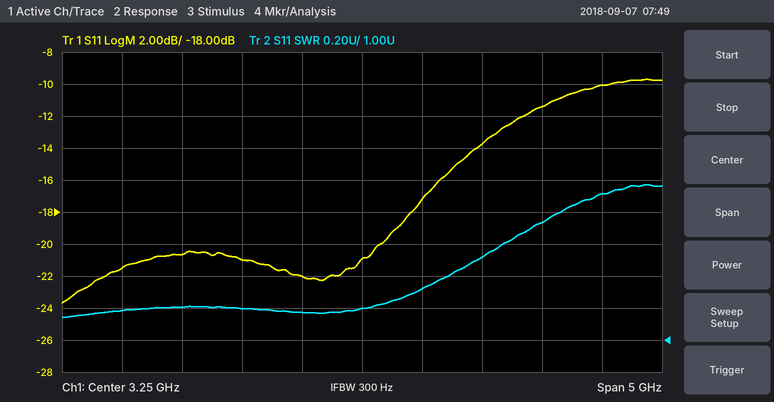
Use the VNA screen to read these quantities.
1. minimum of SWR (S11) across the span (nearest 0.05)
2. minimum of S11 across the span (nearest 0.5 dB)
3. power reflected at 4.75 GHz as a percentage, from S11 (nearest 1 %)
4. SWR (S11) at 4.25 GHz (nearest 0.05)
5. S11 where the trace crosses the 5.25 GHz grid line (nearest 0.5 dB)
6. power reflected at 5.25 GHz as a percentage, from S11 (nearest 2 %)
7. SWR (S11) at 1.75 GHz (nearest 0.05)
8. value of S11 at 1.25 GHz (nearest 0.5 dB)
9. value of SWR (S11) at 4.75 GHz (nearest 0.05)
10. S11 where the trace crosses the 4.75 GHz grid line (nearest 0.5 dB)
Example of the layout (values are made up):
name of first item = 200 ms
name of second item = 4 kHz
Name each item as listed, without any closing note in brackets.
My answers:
minimum of SWR (S11) across the span = 1.15
minimum of S11 across the span = -23.5 dB
power reflected at 4.75 GHz as a percentage, from S11 = 7 %
SWR (S11) at 4.25 GHz = 1.50
S11 where the trace crosses the 5.25 GHz grid line = -10.0 dB
power reflected at 5.25 GHz as a percentage, from S11 = 10 %
SWR (S11) at 1.75 GHz = 1.20
value of S11 at 1.25 GHz = -21.5 dB
value of SWR (S11) at 4.75 GHz = 1.75
S11 where the trace crosses the 4.75 GHz grid line = -11.5 dB
